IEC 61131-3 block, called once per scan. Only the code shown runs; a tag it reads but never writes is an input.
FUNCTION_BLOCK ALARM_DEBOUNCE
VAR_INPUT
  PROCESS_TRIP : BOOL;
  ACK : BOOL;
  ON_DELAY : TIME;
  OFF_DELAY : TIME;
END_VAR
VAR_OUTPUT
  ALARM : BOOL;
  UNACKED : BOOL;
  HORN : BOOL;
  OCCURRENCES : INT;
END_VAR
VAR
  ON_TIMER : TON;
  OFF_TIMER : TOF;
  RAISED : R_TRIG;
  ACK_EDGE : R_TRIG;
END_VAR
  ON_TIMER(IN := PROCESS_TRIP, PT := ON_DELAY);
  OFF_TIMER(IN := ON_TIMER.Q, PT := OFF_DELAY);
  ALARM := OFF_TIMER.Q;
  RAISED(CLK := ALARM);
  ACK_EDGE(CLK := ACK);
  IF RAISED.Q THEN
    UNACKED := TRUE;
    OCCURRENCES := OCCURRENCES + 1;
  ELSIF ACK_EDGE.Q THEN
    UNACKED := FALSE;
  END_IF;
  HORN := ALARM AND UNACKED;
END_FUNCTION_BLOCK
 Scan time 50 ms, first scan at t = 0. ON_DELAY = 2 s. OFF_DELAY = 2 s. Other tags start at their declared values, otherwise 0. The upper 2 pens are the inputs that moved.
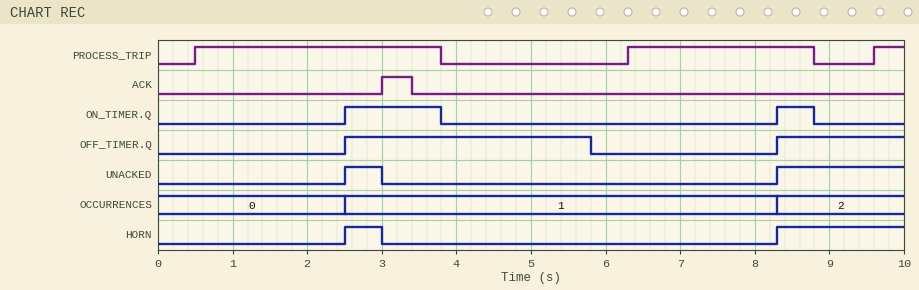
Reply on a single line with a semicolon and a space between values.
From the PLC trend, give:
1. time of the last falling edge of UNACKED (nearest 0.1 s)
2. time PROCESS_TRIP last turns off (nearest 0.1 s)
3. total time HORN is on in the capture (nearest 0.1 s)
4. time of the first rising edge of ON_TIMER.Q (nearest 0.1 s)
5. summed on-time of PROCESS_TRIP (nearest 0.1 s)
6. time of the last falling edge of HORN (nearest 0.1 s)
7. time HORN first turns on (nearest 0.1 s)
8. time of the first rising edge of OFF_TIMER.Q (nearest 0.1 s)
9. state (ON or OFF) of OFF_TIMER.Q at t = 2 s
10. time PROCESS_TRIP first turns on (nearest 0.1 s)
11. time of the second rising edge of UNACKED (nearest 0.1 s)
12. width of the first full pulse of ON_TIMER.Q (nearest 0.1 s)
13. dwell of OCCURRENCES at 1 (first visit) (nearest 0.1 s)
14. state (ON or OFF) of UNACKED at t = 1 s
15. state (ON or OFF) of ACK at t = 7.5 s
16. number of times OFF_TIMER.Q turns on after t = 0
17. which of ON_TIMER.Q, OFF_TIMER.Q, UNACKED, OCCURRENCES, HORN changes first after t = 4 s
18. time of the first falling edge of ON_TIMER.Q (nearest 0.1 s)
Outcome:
3.0 s; 8.8 s; 2.2 s; 2.5 s; 6.2 s; 3.0 s; 2.5 s; 2.5 s; OFF; 0.5 s; 8.3 s; 1.3 s; 5.8 s; OFF; OFF; 2; OFF_TIMER.Q; 3.8 s
